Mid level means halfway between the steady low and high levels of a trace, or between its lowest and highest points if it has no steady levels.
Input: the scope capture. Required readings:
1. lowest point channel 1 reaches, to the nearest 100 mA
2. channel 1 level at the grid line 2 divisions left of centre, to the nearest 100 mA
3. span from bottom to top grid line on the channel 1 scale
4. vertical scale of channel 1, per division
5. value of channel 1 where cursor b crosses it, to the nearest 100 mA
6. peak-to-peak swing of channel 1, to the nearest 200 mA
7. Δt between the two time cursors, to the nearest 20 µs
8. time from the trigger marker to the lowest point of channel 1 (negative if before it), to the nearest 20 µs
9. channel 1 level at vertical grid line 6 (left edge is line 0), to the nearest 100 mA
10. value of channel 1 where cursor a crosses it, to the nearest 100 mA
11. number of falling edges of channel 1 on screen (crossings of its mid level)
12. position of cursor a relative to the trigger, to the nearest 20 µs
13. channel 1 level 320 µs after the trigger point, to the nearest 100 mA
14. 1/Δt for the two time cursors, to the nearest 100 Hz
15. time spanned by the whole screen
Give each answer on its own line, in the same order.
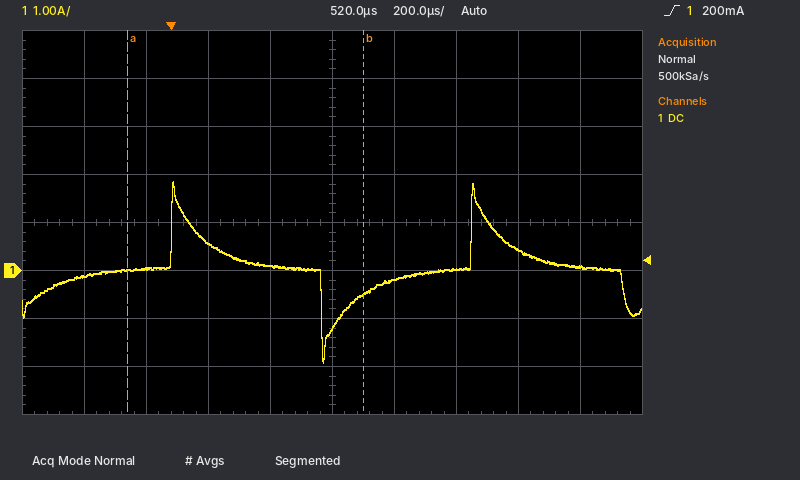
-1.9 A
600 mA
8 A
1 A
-500 mA
3.8 A
760 µs
+500 µs
-200 mA
0.0 A
2
-140 µs
100 mA
1.3 kHz
2 ms
